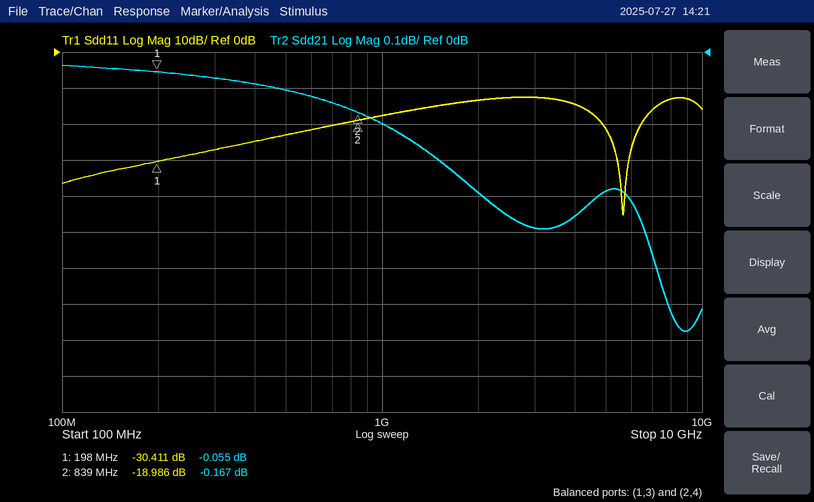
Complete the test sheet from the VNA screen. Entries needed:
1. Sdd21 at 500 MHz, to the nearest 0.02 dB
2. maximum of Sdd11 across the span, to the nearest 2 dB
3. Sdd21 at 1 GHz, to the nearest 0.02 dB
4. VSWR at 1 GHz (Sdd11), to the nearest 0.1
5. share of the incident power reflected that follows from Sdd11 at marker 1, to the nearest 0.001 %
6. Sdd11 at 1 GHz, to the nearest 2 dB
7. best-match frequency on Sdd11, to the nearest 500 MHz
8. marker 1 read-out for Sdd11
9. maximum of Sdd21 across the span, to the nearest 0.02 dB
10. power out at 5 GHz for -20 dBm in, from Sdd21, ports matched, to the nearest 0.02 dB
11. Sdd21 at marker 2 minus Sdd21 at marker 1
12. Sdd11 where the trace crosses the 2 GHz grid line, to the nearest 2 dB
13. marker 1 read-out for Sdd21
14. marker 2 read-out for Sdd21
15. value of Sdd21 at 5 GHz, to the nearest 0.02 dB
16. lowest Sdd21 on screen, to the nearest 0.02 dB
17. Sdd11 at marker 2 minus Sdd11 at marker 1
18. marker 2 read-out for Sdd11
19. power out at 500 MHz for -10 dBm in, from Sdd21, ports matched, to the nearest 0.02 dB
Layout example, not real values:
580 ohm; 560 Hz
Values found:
-0.10 dB; -12 dB; -0.20 dB; 1.3; 0.091 %; -18 dB; 5.5 GHz; -30.411 dB; -0.04 dB; -20.38 dBm; -0.112 dB; -14 dB; -0.055 dB; -0.167 dB; -0.38 dB; -0.78 dB; 11.425 dB; -18.986 dB; -10.10 dBm
